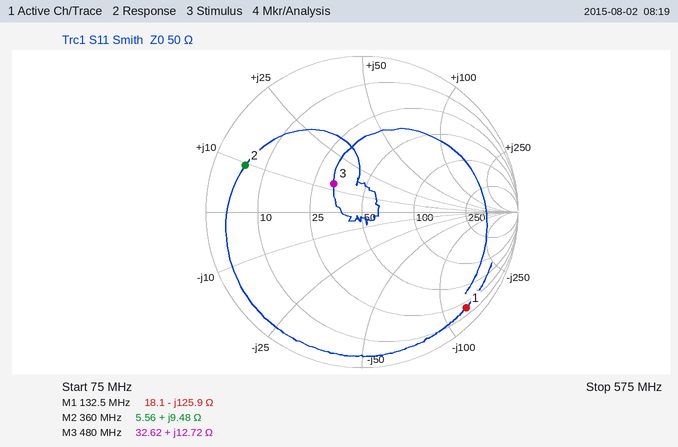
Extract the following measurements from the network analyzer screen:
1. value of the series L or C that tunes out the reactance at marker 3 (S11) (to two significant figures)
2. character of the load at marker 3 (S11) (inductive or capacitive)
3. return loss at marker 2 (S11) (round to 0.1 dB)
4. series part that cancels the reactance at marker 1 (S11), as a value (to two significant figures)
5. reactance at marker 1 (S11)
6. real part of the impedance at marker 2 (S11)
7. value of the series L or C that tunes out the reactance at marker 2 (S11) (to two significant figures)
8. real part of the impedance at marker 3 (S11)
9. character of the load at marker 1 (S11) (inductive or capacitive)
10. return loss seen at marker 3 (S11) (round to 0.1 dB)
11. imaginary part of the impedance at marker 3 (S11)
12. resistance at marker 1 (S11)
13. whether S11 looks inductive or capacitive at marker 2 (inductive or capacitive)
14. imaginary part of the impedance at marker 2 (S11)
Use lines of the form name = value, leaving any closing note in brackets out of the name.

value of the series L or C that tunes out the reactance at marker 3 (S11) = 26 pF
character of the load at marker 3 (S11) = inductive
return loss at marker 2 (S11) = 1.9 dB
series part that cancels the reactance at marker 1 (S11), as a value = 150 nH
reactance at marker 1 = -125.9 Ω
real part of the impedance at marker 2 = 5.56 Ω
value of the series L or C that tunes out the reactance at marker 2 (S11) = 47 pF
real part of the impedance at marker 3 = 32.62 Ω
character of the load at marker 1 (S11) = capacitive
return loss seen at marker 3 (S11) = 11.8 dB
imaginary part of the impedance at marker 3 = +12.72 Ω
resistance at marker 1 = 18.1 Ω
whether S11 looks inductive or capacitive at marker 2 = inductive
imaginary part of the impedance at marker 2 = +9.48 Ω
